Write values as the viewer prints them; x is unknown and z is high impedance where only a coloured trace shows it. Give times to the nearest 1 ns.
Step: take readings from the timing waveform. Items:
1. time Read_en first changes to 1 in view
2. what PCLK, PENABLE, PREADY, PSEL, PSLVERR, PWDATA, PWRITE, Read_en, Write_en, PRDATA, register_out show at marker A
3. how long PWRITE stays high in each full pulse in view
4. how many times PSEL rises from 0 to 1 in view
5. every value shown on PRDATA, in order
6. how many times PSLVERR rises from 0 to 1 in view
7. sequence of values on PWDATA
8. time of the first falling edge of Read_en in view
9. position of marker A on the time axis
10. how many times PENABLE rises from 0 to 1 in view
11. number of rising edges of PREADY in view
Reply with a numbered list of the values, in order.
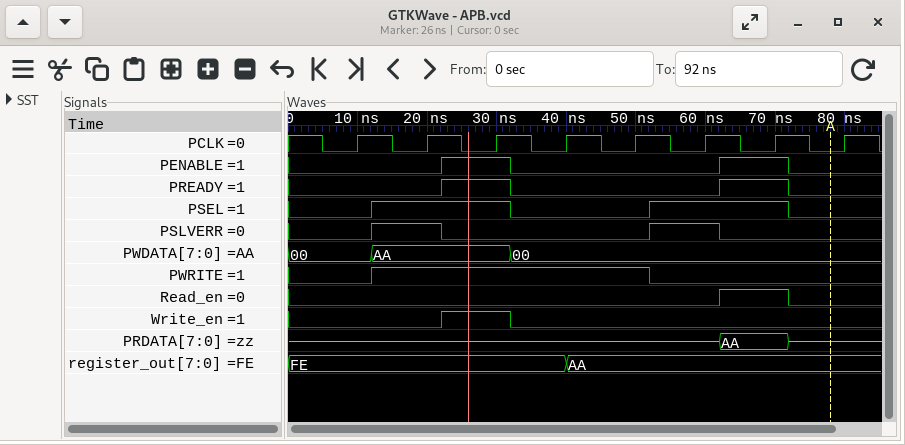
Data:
1. 62 ns
2. PCLK=0, PENABLE=0, PREADY=0, PSEL=0, PSLVERR=0, PWDATA=00, PWRITE=0, Read_en=0, Write_en=0, PRDATA=z, register_out=AA
3. 40 ns
4. 2
5. z, AA, z
6. 2
7. 00, AA, 00
8. 72 ns
9. 78 ns
10. 2
11. 2
